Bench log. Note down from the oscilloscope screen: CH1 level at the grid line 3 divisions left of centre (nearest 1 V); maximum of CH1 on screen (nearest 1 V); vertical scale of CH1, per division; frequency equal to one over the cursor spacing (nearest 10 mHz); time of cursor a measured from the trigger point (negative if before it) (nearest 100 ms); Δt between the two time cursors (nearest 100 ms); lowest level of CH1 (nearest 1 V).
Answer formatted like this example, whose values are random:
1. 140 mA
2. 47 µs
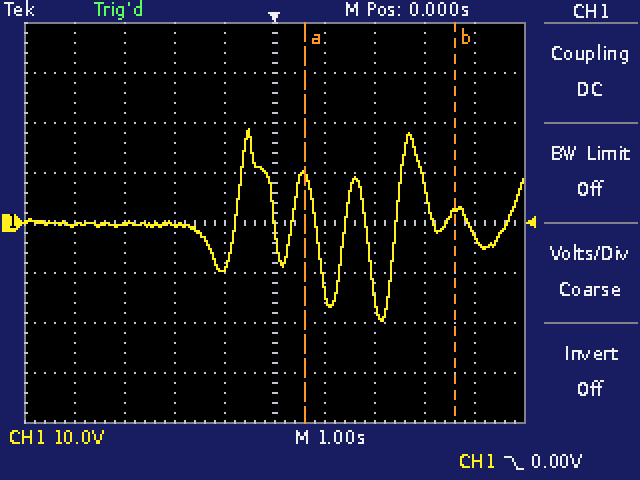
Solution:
1. 0 V
2. 19 V
3. 10 V
4. 330 mHz
5. +600 ms
6. 3.0 s
7. -20 V
